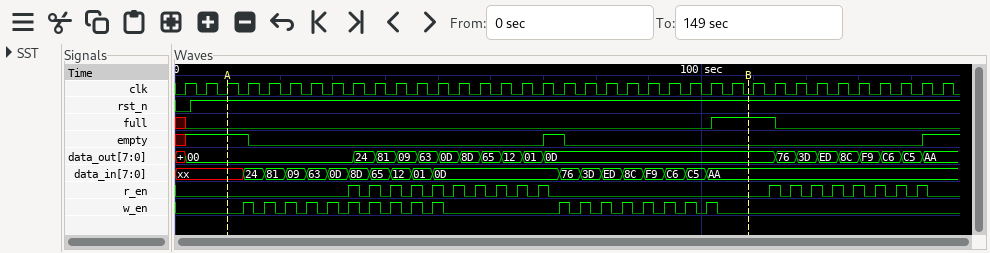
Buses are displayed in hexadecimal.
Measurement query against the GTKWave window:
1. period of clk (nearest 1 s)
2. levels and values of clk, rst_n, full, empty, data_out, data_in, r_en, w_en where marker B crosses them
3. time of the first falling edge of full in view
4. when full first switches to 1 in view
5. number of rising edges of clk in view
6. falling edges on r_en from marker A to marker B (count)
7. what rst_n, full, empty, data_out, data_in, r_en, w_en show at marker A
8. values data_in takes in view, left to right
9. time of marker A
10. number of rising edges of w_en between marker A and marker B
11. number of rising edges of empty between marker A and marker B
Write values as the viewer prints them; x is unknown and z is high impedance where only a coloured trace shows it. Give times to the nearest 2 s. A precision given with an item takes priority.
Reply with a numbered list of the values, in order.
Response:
1. 4 s
2. clk=0, rst_n=1, full=1, empty=0, data_out=0D, data_in=AA, r_en=0, w_en=0
3. 114 s
4. 102 s
5. 37
6. 10
7. rst_n=1, full=0, empty=1, data_out=00, data_in=xx, r_en=0, w_en=0
8. xx, 24, 81, 09, 63, 0D, 8D, 65, 12, 01, 0D, 76, 3D, ED, 8C, F9, C6, C5, AA
9. 10 s
10. 18
11. 1
